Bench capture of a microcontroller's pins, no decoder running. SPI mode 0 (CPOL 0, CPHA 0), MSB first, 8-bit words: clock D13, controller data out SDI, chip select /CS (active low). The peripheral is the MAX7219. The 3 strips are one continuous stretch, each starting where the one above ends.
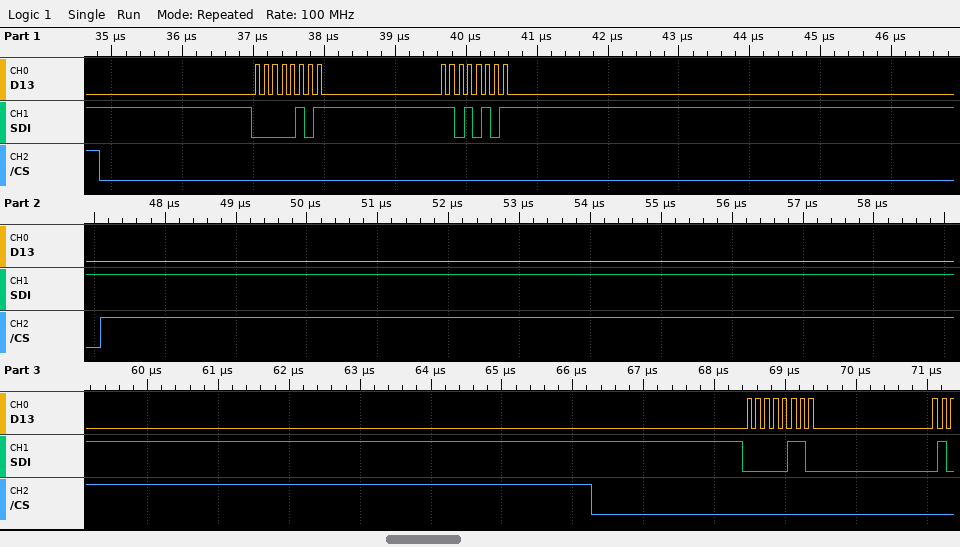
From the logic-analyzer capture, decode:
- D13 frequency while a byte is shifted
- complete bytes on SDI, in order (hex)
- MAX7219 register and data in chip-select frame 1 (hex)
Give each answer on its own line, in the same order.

8 MHz
05 D5 06
register 0x5, data 0xD5
